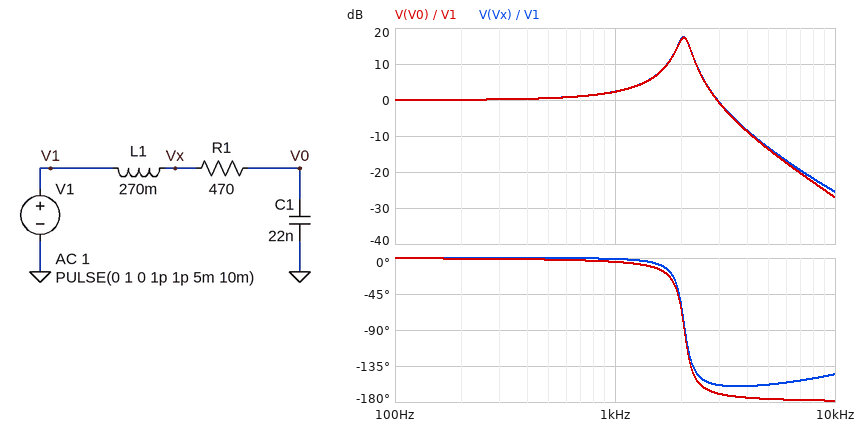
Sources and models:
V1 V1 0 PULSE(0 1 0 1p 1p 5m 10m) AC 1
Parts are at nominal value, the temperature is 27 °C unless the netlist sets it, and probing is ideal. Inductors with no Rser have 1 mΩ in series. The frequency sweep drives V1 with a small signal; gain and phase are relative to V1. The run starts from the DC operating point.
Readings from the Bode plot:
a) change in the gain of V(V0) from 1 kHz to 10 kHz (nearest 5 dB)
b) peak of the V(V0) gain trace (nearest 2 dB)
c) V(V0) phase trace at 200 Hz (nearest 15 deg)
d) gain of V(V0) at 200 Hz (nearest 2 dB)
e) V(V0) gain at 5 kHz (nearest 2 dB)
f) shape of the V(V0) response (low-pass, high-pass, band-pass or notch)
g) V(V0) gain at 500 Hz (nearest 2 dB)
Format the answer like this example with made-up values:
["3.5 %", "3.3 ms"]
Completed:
["-30 dB", "18 dB", "0 deg", "0 dB", "-14 dB", "low-pass", "0 dB"]
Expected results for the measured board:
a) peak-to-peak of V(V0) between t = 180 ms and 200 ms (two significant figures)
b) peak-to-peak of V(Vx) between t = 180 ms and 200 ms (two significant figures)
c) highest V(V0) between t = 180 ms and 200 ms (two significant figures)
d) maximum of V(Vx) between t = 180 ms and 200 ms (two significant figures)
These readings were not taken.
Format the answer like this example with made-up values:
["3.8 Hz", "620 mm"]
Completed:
["2.6 V", "2.6 V", "1.8 V", "1.8 V"]
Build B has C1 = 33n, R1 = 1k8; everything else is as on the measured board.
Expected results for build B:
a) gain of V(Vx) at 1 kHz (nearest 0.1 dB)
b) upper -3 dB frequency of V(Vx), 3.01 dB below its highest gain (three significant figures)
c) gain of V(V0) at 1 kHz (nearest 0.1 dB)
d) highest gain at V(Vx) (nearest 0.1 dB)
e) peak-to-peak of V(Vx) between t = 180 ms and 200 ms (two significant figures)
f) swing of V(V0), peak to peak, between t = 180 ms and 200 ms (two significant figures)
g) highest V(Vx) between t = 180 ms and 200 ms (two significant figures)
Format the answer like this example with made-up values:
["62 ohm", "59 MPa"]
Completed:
["3.1 dB", "2.07 kHz", "2.5 dB", "5.7 dB", "1.9 V", "1.7 V", "1.4 V"]
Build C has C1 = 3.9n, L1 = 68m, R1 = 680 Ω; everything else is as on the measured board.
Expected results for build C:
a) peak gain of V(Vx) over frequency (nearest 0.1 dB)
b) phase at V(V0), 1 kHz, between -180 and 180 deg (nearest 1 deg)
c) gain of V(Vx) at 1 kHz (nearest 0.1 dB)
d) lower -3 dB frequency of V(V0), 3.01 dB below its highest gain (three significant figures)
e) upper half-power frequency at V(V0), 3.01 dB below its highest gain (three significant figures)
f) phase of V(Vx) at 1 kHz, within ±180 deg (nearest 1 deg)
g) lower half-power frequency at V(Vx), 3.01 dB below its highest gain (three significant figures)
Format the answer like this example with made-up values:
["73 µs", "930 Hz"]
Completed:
["15.9 dB", "-1 deg", "0.1 dB", "8.87 kHz", "10.5 kHz", "0 deg", "8.88 kHz"]
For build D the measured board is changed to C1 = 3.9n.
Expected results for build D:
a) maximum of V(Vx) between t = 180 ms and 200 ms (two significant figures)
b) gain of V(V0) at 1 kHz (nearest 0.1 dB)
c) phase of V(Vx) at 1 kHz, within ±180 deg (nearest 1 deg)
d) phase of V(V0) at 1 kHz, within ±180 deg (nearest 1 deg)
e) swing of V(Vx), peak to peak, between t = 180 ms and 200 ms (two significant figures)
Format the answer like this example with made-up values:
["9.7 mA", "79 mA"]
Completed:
["1.9 V", "0.4 dB", "0 deg", "-1 deg", "2.8 V"]
